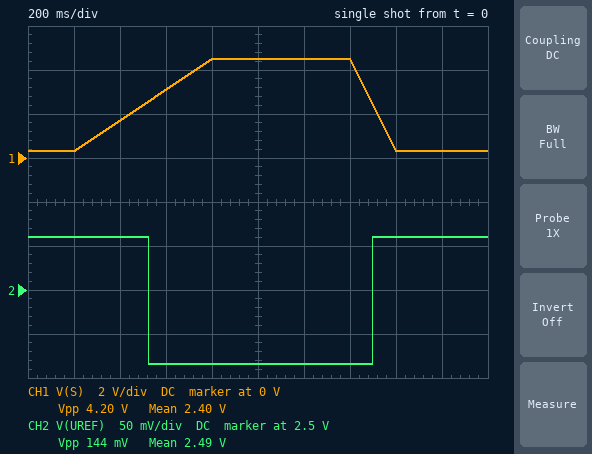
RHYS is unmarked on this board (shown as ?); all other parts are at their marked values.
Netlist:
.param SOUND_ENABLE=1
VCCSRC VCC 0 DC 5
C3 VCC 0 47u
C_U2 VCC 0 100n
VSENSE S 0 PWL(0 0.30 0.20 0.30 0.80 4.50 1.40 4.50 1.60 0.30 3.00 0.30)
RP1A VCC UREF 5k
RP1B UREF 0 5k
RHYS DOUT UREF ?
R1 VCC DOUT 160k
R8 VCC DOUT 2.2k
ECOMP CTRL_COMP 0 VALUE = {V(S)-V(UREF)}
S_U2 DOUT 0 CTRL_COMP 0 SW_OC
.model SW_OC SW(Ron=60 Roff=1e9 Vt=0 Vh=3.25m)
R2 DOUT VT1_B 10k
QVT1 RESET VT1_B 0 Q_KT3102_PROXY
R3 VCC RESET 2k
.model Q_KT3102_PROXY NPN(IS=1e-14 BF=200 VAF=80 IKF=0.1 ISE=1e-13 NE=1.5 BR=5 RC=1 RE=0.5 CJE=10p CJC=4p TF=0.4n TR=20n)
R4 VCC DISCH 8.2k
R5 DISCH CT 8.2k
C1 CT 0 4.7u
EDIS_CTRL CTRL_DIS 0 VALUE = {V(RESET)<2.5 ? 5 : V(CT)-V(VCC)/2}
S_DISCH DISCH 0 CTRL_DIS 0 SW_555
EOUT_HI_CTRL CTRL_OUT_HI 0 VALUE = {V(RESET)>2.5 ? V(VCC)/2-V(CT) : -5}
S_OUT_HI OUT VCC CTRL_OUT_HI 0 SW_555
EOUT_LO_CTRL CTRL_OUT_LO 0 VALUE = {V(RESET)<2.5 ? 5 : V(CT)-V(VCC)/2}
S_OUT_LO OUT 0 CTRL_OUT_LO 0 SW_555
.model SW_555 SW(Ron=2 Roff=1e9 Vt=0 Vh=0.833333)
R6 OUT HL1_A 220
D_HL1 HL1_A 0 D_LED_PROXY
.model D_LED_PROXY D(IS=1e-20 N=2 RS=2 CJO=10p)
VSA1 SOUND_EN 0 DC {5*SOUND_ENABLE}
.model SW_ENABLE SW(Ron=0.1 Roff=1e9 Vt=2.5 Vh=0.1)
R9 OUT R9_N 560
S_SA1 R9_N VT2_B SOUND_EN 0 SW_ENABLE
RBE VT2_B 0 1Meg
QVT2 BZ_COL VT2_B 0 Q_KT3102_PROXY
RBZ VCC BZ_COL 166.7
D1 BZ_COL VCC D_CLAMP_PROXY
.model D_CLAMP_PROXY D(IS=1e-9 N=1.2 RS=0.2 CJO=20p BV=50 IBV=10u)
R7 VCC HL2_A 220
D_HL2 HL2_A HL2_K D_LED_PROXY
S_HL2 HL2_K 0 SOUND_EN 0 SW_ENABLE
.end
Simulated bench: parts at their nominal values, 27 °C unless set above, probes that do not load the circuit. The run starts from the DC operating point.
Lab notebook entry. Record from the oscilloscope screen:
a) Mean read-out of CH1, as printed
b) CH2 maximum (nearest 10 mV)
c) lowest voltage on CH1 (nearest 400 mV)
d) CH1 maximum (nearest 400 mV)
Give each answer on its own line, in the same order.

2.40 V
2.56 V
400 mV
4.4 V
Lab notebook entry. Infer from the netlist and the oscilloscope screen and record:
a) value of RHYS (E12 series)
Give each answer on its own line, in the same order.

68 kΩ
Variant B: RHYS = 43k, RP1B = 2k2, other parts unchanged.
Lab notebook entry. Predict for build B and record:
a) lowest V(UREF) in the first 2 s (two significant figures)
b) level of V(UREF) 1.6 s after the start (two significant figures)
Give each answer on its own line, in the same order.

1.5 V
1.6 V
